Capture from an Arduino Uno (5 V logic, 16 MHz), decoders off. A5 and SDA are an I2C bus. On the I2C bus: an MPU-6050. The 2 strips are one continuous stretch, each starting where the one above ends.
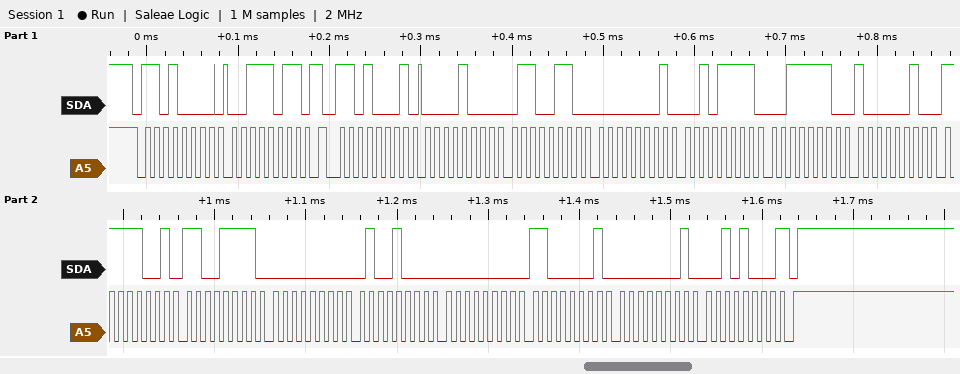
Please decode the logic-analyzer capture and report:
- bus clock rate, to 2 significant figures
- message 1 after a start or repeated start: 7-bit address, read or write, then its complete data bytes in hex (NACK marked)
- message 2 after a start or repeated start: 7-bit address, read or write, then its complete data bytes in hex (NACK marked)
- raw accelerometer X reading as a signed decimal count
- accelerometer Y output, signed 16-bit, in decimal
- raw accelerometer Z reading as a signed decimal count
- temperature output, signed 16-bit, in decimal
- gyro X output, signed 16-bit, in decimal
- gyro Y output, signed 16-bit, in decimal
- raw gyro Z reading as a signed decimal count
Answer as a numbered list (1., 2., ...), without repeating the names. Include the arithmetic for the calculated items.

1. 100 kHz
2. 0x68 write: 3B
3. 0x68 read: 08 66 01 2F 3E 82 F9 CF 00 48 00 C1 01 28 NACK
4. 0x0866 = 2150
5. 0x012F = 303
6. 0x3E82 = 16002
7. 0xF9CF = -1585
8. 0x0048 = 72
9. 0x00C1 = 193
10. 0x0128 = 296
